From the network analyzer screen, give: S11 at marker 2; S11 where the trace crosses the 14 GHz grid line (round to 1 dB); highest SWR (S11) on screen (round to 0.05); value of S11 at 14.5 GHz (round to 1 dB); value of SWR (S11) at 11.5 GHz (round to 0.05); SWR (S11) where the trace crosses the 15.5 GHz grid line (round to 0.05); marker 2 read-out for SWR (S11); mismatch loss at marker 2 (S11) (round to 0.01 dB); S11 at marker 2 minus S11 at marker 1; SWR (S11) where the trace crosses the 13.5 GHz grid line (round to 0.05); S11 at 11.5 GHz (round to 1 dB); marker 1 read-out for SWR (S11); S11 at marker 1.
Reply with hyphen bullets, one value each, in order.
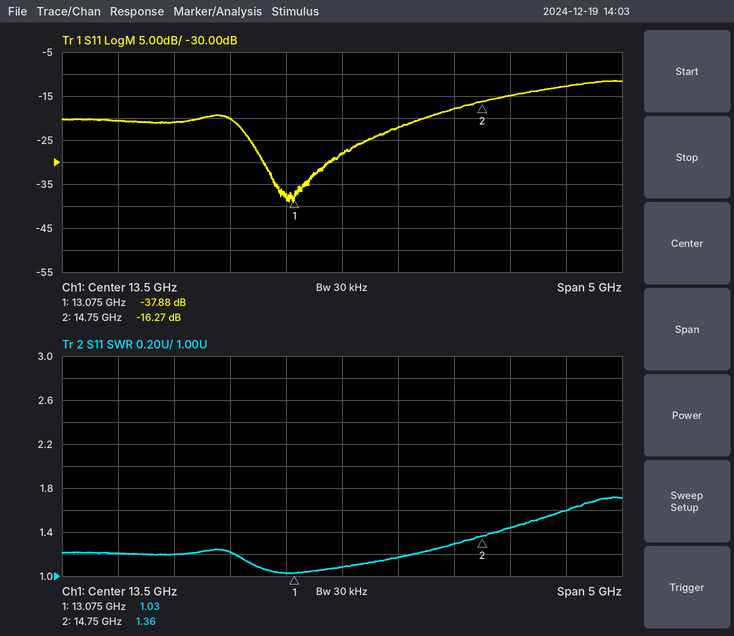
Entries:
- -16.27 dB
- -22 dB
- 1.70
- -18 dB
- 1.20
- 1.60
- 1.36
- 0.10 dB
- 21.61 dB
- 1.10
- -21 dB
- 1.03
- -37.88 dB
